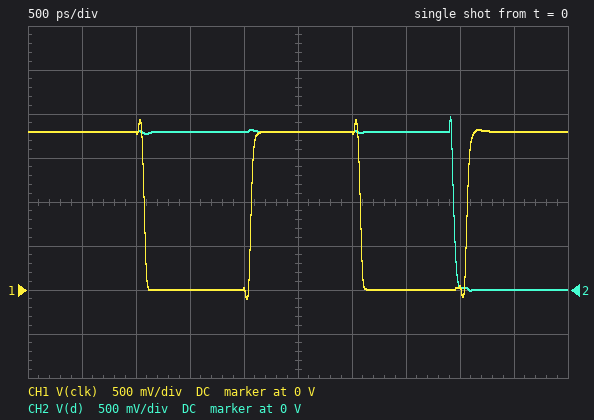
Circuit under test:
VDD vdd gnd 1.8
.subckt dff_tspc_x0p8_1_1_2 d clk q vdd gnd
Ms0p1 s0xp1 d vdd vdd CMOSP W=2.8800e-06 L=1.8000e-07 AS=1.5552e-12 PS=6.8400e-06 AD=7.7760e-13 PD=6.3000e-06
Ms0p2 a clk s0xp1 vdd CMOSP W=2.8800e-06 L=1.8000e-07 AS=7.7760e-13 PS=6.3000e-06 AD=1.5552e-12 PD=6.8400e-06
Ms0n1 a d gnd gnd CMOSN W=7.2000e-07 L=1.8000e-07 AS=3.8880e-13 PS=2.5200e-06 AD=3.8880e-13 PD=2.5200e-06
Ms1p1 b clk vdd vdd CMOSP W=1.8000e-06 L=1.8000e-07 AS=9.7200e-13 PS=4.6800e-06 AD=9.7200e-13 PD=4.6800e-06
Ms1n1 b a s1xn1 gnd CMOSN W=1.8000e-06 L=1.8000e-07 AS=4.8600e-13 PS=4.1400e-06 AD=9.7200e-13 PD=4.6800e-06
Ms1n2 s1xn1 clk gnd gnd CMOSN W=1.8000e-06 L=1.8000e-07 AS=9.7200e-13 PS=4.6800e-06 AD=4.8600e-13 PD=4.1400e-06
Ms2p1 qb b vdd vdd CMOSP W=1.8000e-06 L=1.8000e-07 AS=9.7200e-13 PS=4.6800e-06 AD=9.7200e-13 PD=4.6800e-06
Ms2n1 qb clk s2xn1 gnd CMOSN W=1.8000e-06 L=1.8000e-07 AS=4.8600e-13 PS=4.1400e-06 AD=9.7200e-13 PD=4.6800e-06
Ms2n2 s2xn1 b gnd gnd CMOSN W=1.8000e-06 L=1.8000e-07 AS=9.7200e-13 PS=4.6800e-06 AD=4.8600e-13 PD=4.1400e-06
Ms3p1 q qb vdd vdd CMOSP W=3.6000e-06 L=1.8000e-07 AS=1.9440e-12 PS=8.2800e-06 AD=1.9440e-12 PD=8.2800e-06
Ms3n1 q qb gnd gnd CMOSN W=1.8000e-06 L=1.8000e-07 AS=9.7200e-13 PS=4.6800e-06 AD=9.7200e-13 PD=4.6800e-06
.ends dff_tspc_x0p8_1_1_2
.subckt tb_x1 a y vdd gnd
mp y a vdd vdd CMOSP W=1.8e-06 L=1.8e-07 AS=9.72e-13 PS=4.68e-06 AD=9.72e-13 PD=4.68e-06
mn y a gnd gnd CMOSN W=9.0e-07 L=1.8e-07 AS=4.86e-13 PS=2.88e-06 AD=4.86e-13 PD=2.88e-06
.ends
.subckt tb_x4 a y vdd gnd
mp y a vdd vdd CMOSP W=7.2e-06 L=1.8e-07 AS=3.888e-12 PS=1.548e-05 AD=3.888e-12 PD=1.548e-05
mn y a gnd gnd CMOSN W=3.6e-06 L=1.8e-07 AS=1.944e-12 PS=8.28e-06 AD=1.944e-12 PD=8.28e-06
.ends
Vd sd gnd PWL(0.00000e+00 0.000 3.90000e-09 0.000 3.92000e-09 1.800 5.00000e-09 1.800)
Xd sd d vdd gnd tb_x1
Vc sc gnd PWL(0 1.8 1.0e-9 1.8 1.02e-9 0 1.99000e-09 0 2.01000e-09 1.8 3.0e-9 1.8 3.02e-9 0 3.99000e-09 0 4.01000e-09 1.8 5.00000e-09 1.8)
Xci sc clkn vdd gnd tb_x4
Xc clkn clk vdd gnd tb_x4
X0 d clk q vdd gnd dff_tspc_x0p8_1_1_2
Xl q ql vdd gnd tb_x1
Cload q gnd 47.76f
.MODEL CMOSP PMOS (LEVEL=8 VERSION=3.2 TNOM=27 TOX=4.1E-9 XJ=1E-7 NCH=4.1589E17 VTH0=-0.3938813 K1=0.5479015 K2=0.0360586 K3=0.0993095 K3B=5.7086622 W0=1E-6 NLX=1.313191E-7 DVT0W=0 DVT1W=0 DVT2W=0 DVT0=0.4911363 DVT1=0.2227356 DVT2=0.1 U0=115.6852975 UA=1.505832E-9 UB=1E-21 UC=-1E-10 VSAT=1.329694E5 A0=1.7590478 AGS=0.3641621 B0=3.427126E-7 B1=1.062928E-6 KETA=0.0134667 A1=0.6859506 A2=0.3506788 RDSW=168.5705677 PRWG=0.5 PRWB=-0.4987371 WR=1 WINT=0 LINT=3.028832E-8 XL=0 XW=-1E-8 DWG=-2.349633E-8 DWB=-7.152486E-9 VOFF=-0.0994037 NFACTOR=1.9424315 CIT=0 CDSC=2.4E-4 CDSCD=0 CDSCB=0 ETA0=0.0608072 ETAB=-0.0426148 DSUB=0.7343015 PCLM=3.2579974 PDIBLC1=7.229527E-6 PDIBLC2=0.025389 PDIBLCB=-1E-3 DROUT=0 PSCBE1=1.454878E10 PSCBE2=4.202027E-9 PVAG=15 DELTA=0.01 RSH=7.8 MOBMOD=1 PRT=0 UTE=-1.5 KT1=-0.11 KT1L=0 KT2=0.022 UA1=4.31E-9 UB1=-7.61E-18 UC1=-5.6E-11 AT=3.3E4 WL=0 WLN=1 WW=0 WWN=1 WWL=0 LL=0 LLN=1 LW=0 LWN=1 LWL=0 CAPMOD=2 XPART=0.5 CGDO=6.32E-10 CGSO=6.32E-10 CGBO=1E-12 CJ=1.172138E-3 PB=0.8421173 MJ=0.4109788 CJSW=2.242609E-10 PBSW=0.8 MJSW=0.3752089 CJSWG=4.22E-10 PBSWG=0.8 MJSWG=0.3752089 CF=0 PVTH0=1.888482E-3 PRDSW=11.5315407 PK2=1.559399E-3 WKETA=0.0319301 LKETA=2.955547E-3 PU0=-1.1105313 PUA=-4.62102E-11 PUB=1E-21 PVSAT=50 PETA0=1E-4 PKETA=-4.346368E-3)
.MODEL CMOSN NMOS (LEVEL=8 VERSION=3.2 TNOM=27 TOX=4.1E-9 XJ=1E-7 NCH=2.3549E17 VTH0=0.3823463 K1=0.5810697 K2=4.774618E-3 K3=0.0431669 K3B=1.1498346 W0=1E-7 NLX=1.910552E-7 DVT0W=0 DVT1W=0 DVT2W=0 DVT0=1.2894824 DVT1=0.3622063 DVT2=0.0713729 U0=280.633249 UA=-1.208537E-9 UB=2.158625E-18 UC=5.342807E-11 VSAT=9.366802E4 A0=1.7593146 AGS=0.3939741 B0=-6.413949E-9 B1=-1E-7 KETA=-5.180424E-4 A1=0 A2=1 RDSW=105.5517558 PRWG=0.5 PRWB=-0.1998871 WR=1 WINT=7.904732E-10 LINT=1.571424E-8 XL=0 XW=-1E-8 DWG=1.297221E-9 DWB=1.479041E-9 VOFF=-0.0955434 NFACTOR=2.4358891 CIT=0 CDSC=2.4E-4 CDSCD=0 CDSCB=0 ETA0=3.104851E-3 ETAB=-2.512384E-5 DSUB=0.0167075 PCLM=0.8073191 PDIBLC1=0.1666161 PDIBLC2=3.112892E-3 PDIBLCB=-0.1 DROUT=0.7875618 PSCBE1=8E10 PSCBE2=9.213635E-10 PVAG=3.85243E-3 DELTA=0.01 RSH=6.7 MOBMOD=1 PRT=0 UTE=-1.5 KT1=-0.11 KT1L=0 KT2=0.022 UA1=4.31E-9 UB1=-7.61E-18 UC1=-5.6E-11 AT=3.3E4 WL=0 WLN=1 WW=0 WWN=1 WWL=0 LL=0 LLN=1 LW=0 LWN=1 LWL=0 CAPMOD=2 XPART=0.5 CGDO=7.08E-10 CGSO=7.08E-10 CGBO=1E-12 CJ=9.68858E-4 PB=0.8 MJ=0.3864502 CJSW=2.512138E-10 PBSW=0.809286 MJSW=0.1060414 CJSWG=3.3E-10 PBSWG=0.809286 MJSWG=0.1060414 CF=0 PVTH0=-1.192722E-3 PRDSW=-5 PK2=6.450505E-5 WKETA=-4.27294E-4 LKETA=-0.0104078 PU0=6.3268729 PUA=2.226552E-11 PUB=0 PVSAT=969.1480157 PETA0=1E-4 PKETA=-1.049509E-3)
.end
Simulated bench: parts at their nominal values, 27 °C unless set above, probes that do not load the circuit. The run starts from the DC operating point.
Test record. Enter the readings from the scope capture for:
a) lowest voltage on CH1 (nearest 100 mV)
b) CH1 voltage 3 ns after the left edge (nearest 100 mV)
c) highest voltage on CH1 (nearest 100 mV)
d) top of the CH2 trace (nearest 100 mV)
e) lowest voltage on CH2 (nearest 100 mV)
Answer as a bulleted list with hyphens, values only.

- -100 mV
- 1.8 V
- 1.9 V
- 2.0 V
- 0 V
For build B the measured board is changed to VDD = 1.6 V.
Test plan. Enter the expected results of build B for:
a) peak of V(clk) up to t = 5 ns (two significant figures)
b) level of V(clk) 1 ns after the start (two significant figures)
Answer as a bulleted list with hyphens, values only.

- 1.7 V
- 1.6 V
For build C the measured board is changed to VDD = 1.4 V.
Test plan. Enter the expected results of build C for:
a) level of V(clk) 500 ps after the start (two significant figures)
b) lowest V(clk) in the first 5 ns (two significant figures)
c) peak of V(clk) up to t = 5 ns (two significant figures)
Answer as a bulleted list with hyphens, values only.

- 1.4 V
- -150 mV
- 1.5 V
